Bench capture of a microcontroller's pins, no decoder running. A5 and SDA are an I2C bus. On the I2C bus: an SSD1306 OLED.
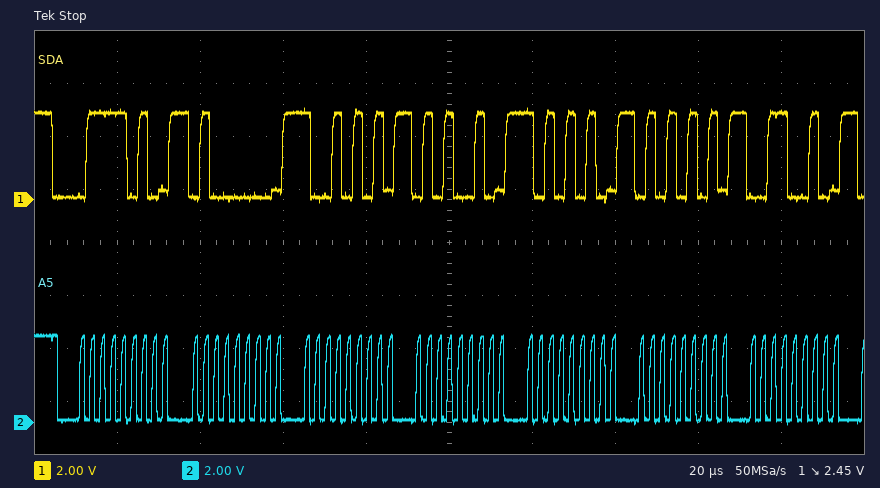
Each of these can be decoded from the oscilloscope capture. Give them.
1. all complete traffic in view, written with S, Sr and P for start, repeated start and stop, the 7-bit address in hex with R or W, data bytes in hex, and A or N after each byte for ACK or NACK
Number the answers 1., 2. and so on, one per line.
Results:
1. S 3DW A 40 A 95 A 52 A AA A 55 A 32 A
